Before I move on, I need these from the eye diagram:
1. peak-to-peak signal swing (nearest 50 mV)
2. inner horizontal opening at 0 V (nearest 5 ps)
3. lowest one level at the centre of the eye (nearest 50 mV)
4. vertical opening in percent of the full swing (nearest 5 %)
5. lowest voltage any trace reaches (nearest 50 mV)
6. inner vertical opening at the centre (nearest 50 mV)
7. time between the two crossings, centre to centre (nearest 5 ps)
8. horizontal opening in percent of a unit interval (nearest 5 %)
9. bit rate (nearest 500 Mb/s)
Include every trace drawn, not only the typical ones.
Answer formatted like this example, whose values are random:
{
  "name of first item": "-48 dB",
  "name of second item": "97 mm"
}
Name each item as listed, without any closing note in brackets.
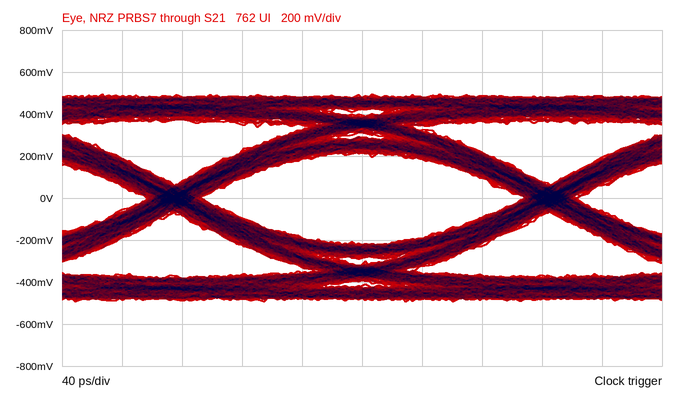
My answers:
{
  "peak-to-peak signal swing": "1.00 V",
  "inner horizontal opening at 0 V": "215 ps",
  "lowest one level at the centre of the eye": "200 mV",
  "vertical opening in percent of the full swing": "45 %",
  "lowest voltage any trace reaches": "-500 mV",
  "inner vertical opening at the centre": "450 mV",
  "time between the two crossings, centre to centre": "250 ps",
  "horizontal opening in percent of a unit interval": "85 %",
  "bit rate": "4.0 Gb/s"
}
